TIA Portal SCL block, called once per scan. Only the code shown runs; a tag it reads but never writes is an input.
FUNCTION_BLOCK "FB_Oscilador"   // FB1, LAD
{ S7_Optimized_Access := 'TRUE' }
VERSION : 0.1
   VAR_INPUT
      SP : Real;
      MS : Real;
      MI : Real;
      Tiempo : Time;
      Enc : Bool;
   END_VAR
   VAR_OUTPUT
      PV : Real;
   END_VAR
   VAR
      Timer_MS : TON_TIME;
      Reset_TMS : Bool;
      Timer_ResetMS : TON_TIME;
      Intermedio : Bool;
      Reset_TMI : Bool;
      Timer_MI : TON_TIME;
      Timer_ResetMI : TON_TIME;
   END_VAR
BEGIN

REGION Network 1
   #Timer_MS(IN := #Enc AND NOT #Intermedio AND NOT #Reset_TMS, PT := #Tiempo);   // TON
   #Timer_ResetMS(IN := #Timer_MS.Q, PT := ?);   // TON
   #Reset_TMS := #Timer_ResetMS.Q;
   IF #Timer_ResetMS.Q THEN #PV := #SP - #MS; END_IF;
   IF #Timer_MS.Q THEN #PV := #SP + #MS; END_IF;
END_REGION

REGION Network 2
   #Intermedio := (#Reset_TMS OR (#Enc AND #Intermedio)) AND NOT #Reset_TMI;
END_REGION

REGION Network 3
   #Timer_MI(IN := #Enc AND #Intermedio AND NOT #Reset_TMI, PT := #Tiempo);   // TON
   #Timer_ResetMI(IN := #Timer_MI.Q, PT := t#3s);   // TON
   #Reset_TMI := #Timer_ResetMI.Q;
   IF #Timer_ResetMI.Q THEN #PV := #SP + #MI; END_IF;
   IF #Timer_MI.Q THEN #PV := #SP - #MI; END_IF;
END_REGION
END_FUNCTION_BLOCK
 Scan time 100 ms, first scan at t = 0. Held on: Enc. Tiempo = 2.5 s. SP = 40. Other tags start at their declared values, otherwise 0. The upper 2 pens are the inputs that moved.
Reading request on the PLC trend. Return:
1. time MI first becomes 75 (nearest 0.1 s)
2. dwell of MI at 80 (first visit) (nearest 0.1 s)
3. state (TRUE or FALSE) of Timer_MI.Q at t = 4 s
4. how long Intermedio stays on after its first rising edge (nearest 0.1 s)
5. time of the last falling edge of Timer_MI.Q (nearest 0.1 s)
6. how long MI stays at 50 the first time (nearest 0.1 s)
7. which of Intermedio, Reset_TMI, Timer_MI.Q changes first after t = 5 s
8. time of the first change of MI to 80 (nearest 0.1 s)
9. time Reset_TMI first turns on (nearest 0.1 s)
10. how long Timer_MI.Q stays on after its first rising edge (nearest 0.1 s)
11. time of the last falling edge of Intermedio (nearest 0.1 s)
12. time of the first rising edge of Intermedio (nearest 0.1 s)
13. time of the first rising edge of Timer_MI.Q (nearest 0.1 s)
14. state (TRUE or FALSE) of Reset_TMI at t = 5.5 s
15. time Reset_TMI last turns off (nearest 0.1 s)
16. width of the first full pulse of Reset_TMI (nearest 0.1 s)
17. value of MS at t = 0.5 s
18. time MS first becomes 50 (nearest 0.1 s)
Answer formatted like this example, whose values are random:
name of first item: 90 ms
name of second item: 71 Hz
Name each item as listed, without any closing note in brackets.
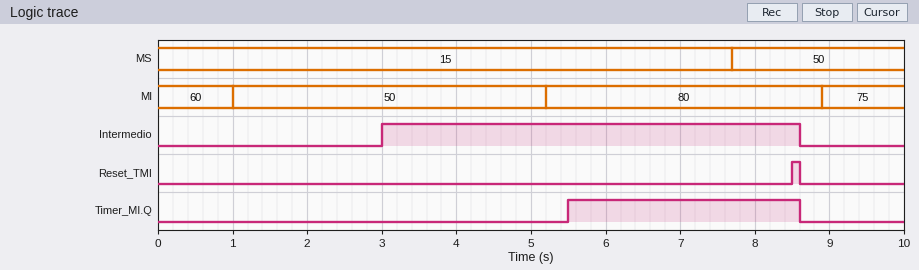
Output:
time MI first becomes 75: 8.9 s
dwell of MI at 80 (first visit): 3.7 s
state (TRUE or FALSE) of Timer_MI.Q at t = 4 s: FALSE
how long Intermedio stays on after its first rising edge: 5.6 s
time of the last falling edge of Timer_MI.Q: 8.6 s
how long MI stays at 50 the first time: 4.2 s
which of Intermedio, Reset_TMI, Timer_MI.Q changes first after t = 5 s: Timer_MI.Q
time of the first change of MI to 80: 5.2 s
time Reset_TMI first turns on: 8.5 s
how long Timer_MI.Q stays on after its first rising edge: 3.1 s
time of the last falling edge of Intermedio: 8.6 s
time of the first rising edge of Intermedio: 3.0 s
time of the first rising edge of Timer_MI.Q: 5.5 s
state (TRUE or FALSE) of Reset_TMI at t = 5.5 s: FALSE
time Reset_TMI last turns off: 8.6 s
width of the first full pulse of Reset_TMI: 0.1 s
value of MS at t = 0.5 s: 15
time MS first becomes 50: 7.7 s
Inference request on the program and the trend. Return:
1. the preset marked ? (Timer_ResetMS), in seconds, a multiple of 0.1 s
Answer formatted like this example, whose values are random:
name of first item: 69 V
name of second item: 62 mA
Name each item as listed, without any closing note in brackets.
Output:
the preset marked ? (Timer_ResetMS), in seconds, a multiple of 0.1 s: 0.5 s
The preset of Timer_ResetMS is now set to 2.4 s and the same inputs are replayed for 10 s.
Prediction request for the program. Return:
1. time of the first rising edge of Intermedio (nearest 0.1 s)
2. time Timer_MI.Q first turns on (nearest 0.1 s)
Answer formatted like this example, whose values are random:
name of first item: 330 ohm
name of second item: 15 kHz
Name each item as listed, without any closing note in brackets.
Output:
time of the first rising edge of Intermedio: 4.9 s
time Timer_MI.Q first turns on: 7.4 s
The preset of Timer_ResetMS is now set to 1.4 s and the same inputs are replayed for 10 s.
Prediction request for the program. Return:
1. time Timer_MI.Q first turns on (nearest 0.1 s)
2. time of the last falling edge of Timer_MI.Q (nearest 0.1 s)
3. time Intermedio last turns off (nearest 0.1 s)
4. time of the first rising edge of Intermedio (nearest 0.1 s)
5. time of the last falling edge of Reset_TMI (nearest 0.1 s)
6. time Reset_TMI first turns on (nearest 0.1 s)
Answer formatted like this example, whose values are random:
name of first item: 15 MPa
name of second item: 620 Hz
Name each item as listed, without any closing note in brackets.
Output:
time Timer_MI.Q first turns on: 6.4 s
time of the last falling edge of Timer_MI.Q: 9.5 s
time Intermedio last turns off: 9.5 s
time of the first rising edge of Intermedio: 3.9 s
time of the last falling edge of Reset_TMI: 9.5 s
time Reset_TMI first turns on: 9.4 s
